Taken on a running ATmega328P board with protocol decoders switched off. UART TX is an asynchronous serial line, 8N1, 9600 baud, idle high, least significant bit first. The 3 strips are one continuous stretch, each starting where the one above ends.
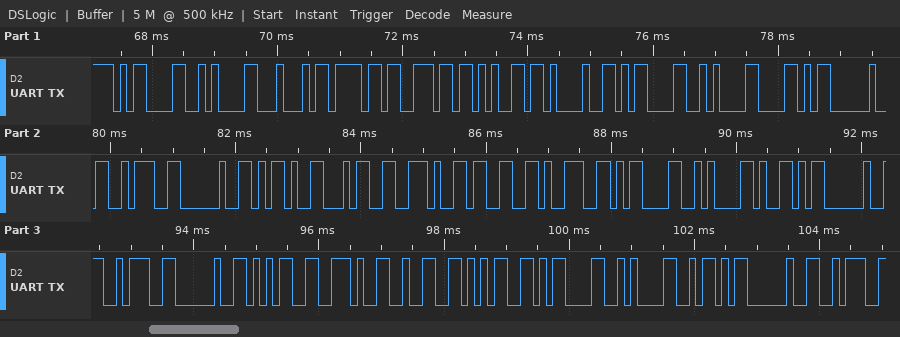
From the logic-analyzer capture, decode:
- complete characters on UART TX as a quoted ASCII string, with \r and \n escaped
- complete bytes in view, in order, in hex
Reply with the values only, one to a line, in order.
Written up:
"\r\nDone!\r\nX : -4.39\r\nY : 5.25\r\nZ :"
0x0D 0x0A 0x44 0x6F 0x6E 0x65 0x21 0x0D 0x0A 0x58 0x20 0x3A 0x20 0x2D 0x34 0x2E 0x33 0x39 0x0D 0x0A 0x59 0x20 0x3A 0x20 0x35 0x2E 0x32 0x35 0x0D 0x0A 0x5A 0x20 0x3A
